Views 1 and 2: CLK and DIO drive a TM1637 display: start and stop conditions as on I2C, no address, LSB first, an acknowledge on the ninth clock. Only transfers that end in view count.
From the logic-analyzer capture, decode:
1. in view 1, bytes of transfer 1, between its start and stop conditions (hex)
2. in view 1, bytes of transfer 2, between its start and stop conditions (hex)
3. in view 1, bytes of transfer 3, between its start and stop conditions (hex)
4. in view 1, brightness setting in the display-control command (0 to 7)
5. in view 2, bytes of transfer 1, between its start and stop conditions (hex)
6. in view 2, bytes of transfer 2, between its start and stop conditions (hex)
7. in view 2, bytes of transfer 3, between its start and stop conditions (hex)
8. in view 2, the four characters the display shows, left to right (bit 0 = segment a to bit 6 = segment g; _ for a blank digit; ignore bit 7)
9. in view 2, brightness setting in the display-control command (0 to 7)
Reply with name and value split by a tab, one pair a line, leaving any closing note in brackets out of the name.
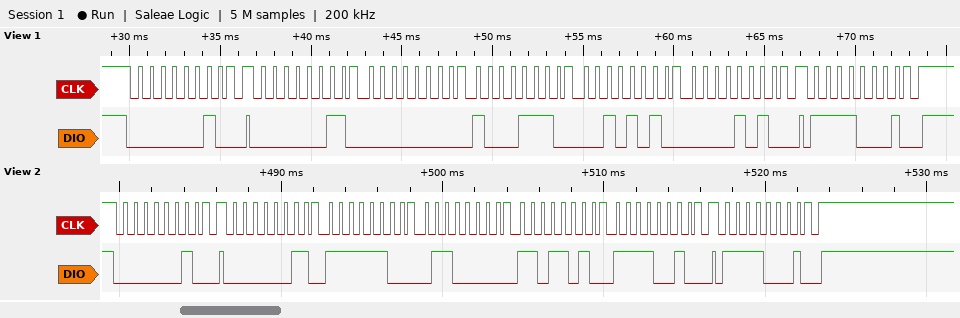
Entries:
in view 1, bytes of transfer 1, between its start and stop conditions	40
in view 1, bytes of transfer 2, between its start and stop conditions	C0 00 71 54 50
in view 1, bytes of transfer 3, between its start and stop conditions	8F
in view 1, brightness setting in the display-control command	7
in view 2, bytes of transfer 1, between its start and stop conditions	40
in view 2, bytes of transfer 2, between its start and stop conditions	C0 3F 06 5B 4F
in view 2, bytes of transfer 3, between its start and stop conditions	8F
in view 2, the four characters the display shows, left to right	0123
in view 2, brightness setting in the display-control command	7
